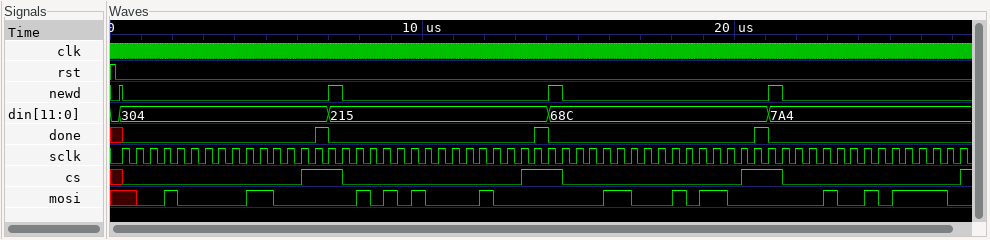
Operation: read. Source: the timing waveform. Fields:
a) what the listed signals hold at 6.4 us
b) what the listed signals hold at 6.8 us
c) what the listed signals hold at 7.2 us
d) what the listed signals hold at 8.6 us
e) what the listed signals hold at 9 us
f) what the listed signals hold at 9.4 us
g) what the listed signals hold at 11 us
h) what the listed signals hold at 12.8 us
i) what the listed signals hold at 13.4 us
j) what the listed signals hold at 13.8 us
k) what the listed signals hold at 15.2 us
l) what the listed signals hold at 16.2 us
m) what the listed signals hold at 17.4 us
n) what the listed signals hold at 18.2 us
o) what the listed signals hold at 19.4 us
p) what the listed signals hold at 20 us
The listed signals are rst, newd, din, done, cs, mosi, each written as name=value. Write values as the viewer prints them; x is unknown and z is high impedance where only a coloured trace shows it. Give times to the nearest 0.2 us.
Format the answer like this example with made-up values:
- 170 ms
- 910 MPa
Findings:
- rst=0, newd=0, din=304, done=0, cs=1, mosi=0
- rst=0, newd=0, din=304, done=1, cs=1, mosi=0
- rst=0, newd=1, din=215, done=0, cs=1, mosi=0
- rst=0, newd=0, din=215, done=0, cs=0, mosi=0
- rst=0, newd=0, din=215, done=0, cs=0, mosi=1
- rst=0, newd=0, din=215, done=0, cs=0, mosi=0
- rst=0, newd=0, din=215, done=0, cs=0, mosi=0
- rst=0, newd=0, din=215, done=0, cs=0, mosi=0
- rst=0, newd=0, din=215, done=0, cs=1, mosi=0
- rst=0, newd=0, din=215, done=1, cs=1, mosi=0
- rst=0, newd=0, din=68C, done=0, cs=0, mosi=0
- rst=0, newd=0, din=68C, done=0, cs=0, mosi=1
- rst=0, newd=0, din=68C, done=0, cs=0, mosi=0
- rst=0, newd=0, din=68C, done=0, cs=0, mosi=1
- rst=0, newd=0, din=68C, done=0, cs=0, mosi=1
- rst=0, newd=0, din=68C, done=0, cs=0, mosi=0
